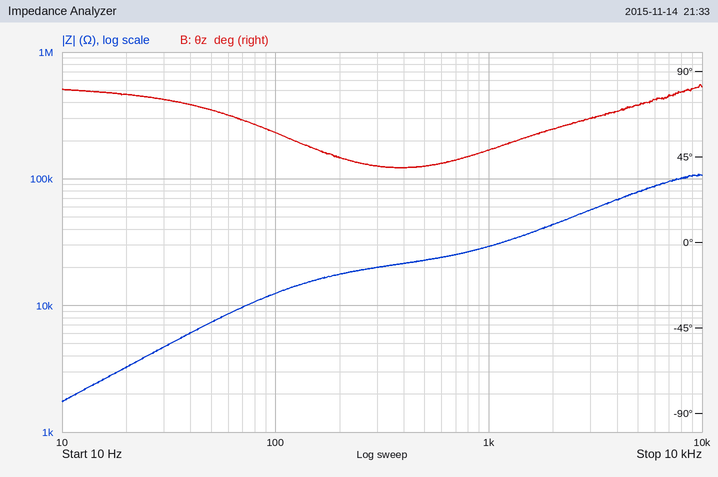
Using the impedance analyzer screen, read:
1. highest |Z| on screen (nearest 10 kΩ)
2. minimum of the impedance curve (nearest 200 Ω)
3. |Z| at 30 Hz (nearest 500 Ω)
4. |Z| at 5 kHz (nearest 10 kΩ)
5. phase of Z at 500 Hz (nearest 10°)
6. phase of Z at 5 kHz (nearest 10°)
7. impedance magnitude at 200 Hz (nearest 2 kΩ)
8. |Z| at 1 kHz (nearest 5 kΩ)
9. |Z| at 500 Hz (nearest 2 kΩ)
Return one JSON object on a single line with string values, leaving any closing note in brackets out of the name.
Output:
{"highest |Z| on screen": "110 kΩ", "minimum of the impedance curve": "1.8 kΩ", "|Z| at 30 Hz": "4.5 kΩ", "|Z| at 5 kHz": "80 kΩ", "phase of Z at 500 Hz": "40°", "phase of Z at 5 kHz": "70°", "impedance magnitude at 200 Hz": "18 kΩ", "|Z| at 1 kHz": "30 kΩ", "|Z| at 500 Hz": "22 kΩ"}
